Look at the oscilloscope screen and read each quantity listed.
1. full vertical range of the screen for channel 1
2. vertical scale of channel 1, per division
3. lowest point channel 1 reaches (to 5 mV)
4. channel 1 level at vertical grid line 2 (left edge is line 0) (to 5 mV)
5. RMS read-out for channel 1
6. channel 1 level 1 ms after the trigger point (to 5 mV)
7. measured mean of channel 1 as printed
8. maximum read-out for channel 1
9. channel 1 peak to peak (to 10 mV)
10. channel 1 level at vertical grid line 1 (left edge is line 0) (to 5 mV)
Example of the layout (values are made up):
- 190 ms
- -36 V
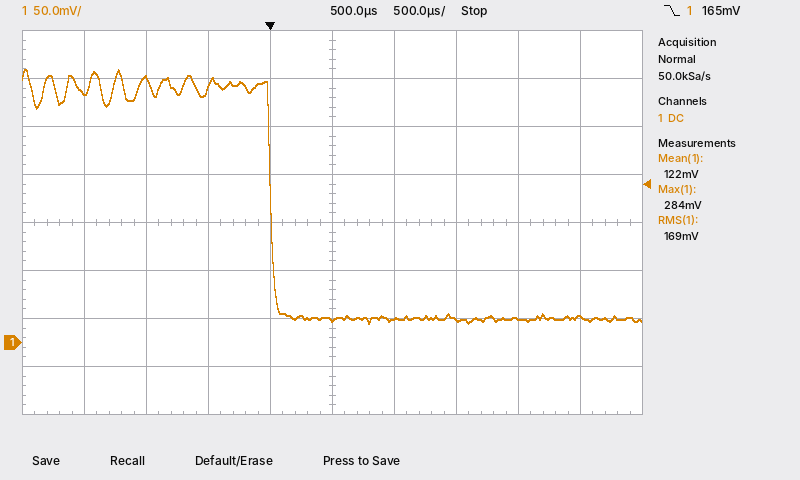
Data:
- 400 mV
- 50 mV
- 20 mV
- 275 mV
- 169 mV
- 25 mV
- 122 mV
- 284 mV
- 260 mV
- 260 mV
